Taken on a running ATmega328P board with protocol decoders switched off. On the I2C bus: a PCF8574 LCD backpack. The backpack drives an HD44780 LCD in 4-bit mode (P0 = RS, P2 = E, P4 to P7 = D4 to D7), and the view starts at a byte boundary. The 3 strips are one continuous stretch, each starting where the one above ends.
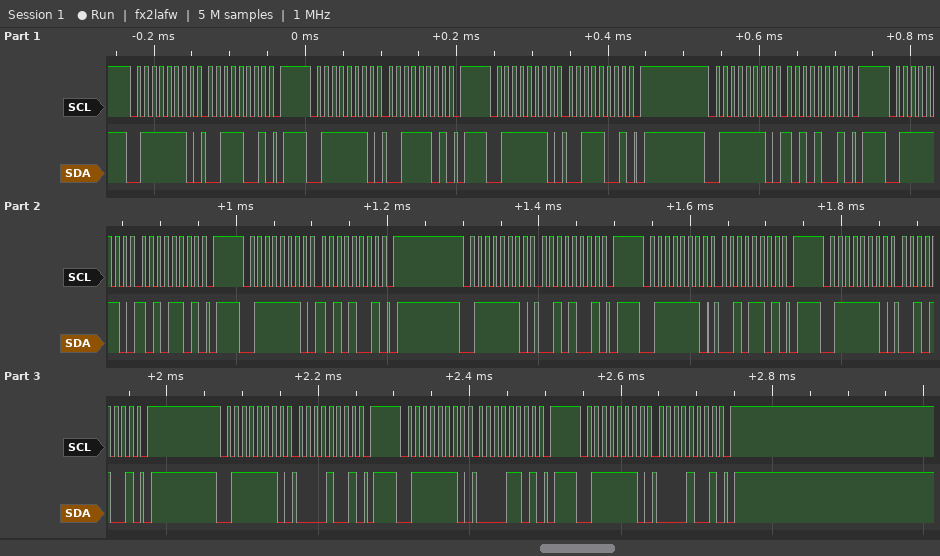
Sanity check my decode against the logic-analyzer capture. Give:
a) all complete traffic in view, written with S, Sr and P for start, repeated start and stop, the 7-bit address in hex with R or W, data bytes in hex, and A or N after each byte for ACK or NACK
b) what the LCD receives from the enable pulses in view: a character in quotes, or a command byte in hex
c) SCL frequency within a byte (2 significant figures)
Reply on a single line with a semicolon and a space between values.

S 3FW A 39 A P S 3FW A 3D A P S 3FW A 39 A P S 3FW A A9 A P S 3FW A AD A P S 3FW A A9 A P S 3FW A 29 A P S 3FW A 2D A P S 3FW A 29 A P S 3FW A 09 A P S 3FW A 0D A P S 3FW A 09 A P; ':' ' '; 100 kHz
